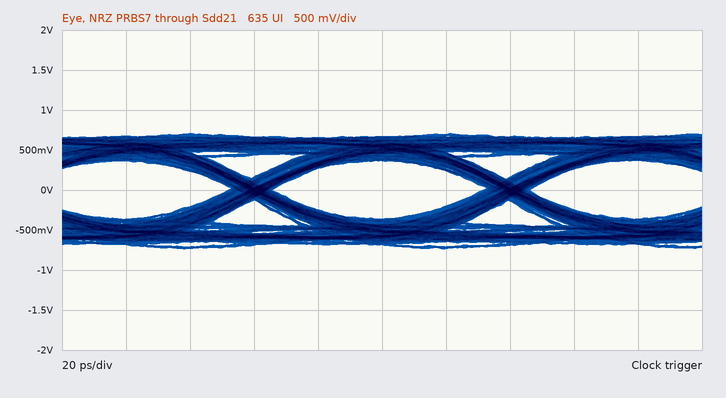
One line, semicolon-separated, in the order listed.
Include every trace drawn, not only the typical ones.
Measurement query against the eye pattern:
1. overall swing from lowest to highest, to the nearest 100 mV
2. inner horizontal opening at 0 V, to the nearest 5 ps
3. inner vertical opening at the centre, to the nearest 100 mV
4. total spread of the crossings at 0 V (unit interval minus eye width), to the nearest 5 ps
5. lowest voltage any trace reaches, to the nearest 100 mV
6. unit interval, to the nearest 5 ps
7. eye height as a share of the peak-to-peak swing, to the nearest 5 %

1.4 V; 65 ps; 700 mV; 15 ps; -700 mV; 80 ps; 50 %
